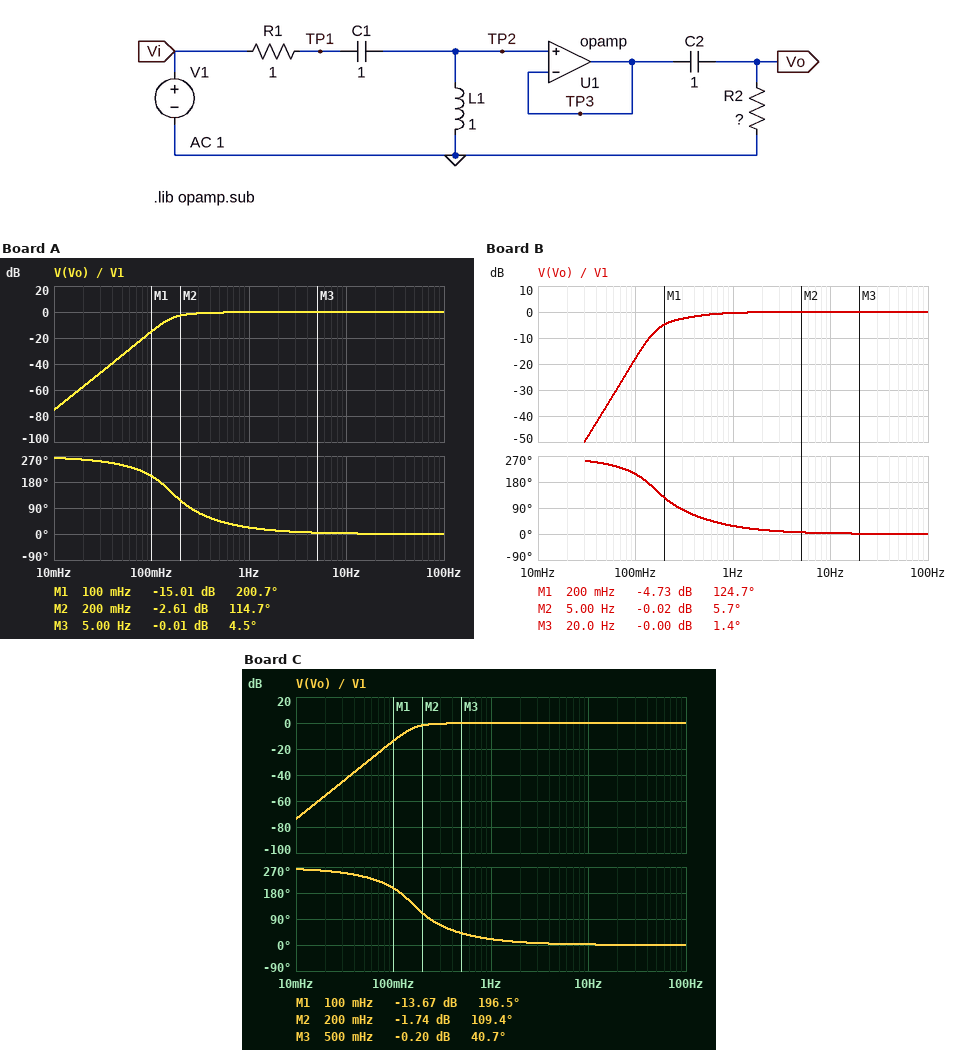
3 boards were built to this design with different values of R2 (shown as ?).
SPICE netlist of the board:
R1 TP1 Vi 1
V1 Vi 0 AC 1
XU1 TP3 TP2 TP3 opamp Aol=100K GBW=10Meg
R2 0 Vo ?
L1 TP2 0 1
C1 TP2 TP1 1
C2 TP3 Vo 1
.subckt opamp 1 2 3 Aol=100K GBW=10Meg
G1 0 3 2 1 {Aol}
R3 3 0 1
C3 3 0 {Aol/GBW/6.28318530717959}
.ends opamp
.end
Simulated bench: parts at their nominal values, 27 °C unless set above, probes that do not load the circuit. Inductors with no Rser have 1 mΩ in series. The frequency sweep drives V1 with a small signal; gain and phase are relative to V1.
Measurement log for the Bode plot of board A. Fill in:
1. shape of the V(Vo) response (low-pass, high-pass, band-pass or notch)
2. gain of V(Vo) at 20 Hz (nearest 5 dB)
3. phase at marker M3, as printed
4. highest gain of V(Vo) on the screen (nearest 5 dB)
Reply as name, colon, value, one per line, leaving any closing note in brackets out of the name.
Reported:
shape of the V(Vo) response: high-pass
gain of V(Vo) at 20 Hz: 0 dB
phase at marker M3, as printed: 4.5 deg
highest gain of V(Vo) on the screen: 0 dB
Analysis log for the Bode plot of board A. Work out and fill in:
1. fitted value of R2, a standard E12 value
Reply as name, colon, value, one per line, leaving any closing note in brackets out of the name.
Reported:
fitted value of R2, a standard E12 value: 0.68 Ω
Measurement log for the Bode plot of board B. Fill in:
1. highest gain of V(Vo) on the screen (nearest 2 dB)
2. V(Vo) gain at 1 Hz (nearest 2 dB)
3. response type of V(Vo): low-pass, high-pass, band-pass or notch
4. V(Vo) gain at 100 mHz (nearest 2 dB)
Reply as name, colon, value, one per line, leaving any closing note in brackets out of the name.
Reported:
highest gain of V(Vo) on the screen: 0 dB
V(Vo) gain at 1 Hz: 0 dB
response type of V(Vo): low-pass, high-pass, band-pass or notch: high-pass
V(Vo) gain at 100 mHz: -18 dB
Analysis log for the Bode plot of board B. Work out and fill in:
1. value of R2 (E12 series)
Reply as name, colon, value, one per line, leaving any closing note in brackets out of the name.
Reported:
value of R2: 0.47 Ω
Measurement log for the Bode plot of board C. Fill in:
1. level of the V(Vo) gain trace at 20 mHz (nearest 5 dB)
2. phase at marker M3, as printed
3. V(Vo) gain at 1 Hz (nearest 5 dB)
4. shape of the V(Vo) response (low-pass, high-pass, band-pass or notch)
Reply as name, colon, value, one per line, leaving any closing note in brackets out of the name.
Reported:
level of the V(Vo) gain trace at 20 mHz: -55 dB
phase at marker M3, as printed: 40.7 deg
V(Vo) gain at 1 Hz: 0 dB
shape of the V(Vo) response: high-pass
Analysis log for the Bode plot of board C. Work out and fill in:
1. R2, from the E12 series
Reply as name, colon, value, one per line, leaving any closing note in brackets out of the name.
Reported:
R2, from the E12 series: 0.82 Ω
